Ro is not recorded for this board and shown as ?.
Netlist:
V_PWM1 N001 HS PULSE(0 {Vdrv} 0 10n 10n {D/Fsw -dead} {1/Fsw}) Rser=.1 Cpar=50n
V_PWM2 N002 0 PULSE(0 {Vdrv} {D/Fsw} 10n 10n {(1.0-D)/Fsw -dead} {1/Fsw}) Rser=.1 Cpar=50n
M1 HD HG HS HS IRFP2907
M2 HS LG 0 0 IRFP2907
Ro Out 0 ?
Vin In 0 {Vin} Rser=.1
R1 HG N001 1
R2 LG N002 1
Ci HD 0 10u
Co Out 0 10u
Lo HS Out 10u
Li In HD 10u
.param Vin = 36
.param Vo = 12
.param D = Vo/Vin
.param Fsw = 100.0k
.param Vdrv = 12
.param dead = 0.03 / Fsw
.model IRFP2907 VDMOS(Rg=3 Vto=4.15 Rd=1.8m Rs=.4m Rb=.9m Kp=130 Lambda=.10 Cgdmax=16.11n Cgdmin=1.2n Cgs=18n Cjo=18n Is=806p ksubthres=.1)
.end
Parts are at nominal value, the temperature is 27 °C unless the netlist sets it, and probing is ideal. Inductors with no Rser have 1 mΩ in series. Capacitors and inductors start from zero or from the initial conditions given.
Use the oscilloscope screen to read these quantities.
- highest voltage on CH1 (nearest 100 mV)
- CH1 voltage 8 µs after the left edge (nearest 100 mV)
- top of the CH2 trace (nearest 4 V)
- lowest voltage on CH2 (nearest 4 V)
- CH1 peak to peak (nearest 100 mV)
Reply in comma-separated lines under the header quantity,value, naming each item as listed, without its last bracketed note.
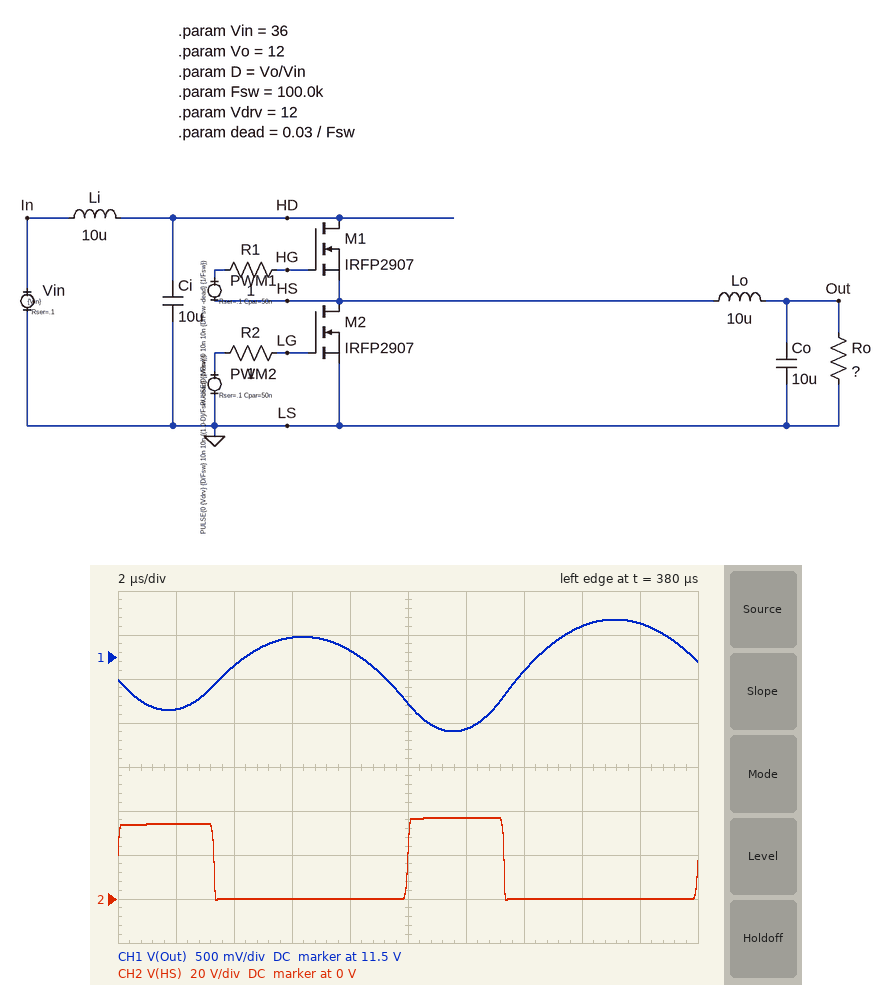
quantity,value
highest voltage on CH1,11.9 V
CH1 voltage 8 µs after the left edge,11.6 V
top of the CH2 trace,36 V
lowest voltage on CH2,0 V
CH1 peak to peak,1.3 V
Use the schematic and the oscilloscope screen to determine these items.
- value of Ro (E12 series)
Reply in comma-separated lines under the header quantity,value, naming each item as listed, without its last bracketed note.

quantity,value
value of Ro,12 Ω
